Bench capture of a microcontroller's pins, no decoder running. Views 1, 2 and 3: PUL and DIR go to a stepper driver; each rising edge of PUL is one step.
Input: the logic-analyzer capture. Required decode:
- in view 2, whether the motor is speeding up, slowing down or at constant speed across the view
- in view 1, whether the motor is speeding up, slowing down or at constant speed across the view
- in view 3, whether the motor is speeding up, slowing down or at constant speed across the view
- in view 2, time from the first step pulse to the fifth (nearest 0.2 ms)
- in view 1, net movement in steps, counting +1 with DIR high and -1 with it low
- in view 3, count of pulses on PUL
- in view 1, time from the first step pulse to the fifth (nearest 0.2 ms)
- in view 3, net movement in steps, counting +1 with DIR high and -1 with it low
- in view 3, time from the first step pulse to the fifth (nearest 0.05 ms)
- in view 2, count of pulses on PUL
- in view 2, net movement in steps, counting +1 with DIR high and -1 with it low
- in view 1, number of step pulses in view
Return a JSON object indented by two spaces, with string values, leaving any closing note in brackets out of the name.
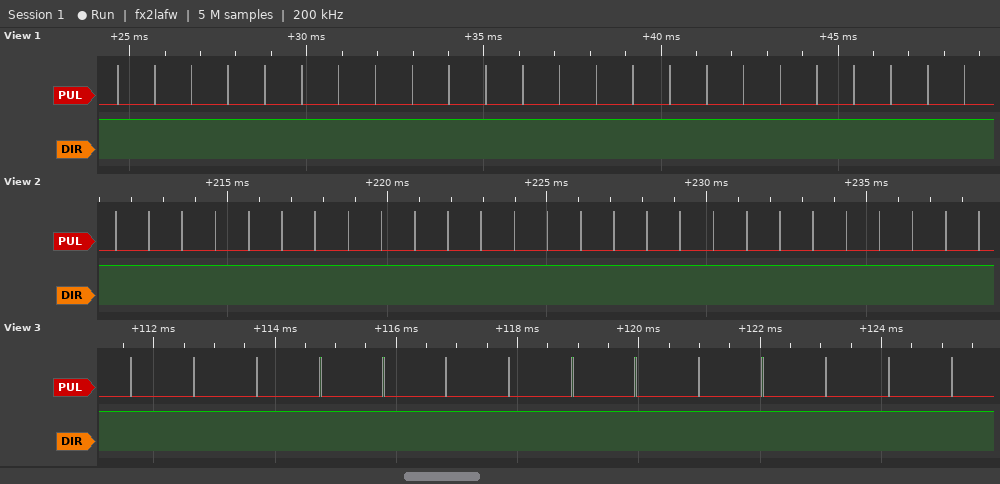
{
  "in view 2, whether the motor is speeding up, slowing down or at constant speed across the view": "constant speed",
  "in view 1, whether the motor is speeding up, slowing down or at constant speed across the view": "constant speed",
  "in view 3, whether the motor is speeding up, slowing down or at constant speed across the view": "constant speed",
  "in view 2, time from the first step pulse to the fifth": "4.2 ms",
  "in view 1, net movement in steps, counting +1 with DIR high and -1 with it low": "+24",
  "in view 3, count of pulses on PUL": "14",
  "in view 1, time from the first step pulse to the fifth": "4.2 ms",
  "in view 3, net movement in steps, counting +1 with DIR high and -1 with it low": "+14",
  "in view 3, time from the first step pulse to the fifth": "4.15 ms",
  "in view 2, count of pulses on PUL": "27",
  "in view 2, net movement in steps, counting +1 with DIR high and -1 with it low": "+27",
  "in view 1, number of step pulses in view": "24"
}
